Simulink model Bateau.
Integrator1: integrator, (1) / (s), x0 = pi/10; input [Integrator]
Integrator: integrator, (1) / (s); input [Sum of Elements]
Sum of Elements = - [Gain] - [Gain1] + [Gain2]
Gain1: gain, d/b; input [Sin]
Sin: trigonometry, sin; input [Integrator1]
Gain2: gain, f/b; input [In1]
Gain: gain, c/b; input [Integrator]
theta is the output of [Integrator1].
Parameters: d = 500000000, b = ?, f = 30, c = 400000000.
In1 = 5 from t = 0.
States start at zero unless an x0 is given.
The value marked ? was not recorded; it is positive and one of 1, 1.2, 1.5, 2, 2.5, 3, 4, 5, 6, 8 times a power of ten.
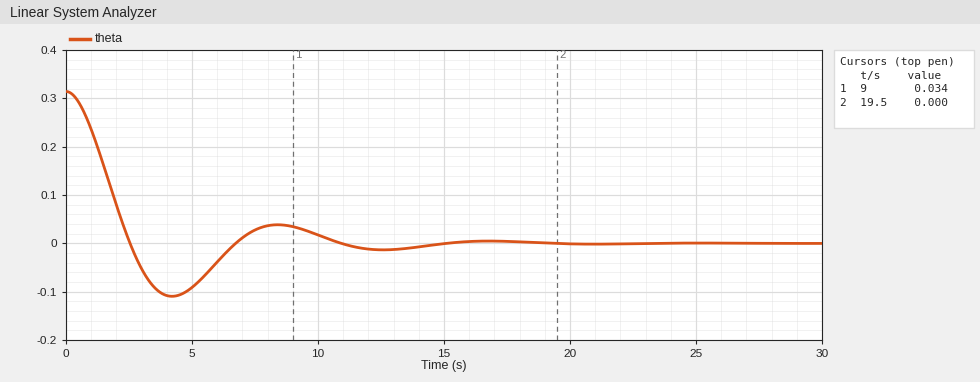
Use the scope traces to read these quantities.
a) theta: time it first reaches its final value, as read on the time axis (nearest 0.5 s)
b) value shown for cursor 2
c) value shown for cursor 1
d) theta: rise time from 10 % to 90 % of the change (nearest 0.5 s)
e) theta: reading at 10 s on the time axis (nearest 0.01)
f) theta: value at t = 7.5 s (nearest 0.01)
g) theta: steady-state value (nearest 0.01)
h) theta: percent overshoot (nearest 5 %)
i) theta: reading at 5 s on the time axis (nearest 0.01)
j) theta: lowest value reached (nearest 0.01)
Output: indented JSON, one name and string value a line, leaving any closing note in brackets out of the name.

{
  "theta: time it first reaches its final value, as read on the time axis": "2.5 s",
  "value shown for cursor 2": "0.000",
  "value shown for cursor 1": "0.034",
  "theta: rise time from 10 % to 90 % of the change": "1.5 s",
  "theta: reading at 10 s on the time axis": "0.02",
  "theta: value at t = 7.5 s": "0.03",
  "theta: steady-state value": "0.00",
  "theta: percent overshoot": "35 %",
  "theta: reading at 5 s on the time axis": "-0.09",
  "theta: lowest value reached": "-0.11"
}
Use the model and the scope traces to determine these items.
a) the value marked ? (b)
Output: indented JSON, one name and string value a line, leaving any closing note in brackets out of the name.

{
  "the value marked ?": "8e+08"
}
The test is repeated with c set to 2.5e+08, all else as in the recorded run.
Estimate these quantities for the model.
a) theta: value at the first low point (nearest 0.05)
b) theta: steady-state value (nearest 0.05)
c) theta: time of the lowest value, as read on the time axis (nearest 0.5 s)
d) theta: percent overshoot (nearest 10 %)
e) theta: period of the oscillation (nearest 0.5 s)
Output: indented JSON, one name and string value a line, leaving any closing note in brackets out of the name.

{
  "theta: value at the first low point": "-0.15",
  "theta: steady-state value": "0.00",
  "theta: time of the lowest value, as read on the time axis": "4.0 s",
  "theta: percent overshoot": "50 %",
  "theta: period of the oscillation": "8.0 s"
}
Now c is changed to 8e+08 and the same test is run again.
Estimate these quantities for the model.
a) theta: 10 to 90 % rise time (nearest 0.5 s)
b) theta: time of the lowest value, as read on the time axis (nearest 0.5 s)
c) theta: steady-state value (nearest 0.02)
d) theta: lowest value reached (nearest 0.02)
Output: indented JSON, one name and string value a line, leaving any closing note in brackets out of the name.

{
  "theta: 10 to 90 % rise time": "2.5 s",
  "theta: time of the lowest value, as read on the time axis": "5.0 s",
  "theta: steady-state value": "0.00",
  "theta: lowest value reached": "-0.02"
}
